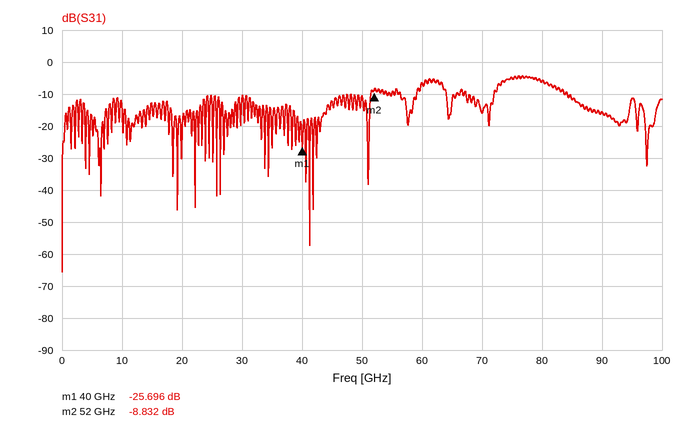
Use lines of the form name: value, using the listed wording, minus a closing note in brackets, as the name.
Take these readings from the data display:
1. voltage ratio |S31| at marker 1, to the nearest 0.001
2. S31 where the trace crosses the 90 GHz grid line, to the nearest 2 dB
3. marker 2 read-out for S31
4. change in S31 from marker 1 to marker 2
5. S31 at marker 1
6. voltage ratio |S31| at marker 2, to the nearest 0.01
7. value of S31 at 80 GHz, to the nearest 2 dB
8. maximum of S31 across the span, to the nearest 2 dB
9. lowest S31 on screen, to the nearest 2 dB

voltage ratio |S31| at marker 1, to the nearest 0.001: 0.052
S31 where the trace crosses the 90 GHz grid line, to the nearest 2 dB: -16 dB
marker 2 read-out for S31: -8.832 dB
change in S31 from marker 1 to marker 2: 16.864 dB
S31 at marker 1: -25.696 dB
voltage ratio |S31| at marker 2, to the nearest 0.01: 0.36
value of S31 at 80 GHz, to the nearest 2 dB: -6 dB
maximum of S31 across the span, to the nearest 2 dB: -4 dB
lowest S31 on screen, to the nearest 2 dB: -66 dB
